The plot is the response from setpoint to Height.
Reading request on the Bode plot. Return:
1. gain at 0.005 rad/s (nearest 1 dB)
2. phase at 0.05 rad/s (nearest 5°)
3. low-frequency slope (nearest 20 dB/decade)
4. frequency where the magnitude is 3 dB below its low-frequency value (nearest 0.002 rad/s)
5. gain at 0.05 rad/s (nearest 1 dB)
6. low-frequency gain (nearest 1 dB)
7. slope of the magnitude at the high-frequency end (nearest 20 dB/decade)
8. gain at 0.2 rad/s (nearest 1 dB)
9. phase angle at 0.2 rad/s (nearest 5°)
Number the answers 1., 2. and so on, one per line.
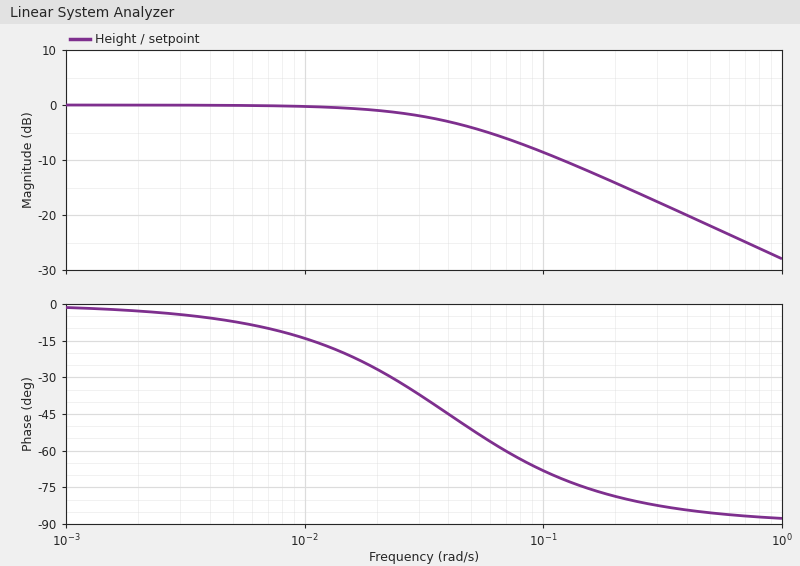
1. 0 dB
2. -50°
3. 0 dB/decade
4. 0.040 rad/s
5. -4 dB
6. 0 dB
7. -20 dB/decade
8. -14 dB
9. -80°
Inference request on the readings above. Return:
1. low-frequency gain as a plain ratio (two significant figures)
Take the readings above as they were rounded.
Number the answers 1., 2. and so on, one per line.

1. 1.0
